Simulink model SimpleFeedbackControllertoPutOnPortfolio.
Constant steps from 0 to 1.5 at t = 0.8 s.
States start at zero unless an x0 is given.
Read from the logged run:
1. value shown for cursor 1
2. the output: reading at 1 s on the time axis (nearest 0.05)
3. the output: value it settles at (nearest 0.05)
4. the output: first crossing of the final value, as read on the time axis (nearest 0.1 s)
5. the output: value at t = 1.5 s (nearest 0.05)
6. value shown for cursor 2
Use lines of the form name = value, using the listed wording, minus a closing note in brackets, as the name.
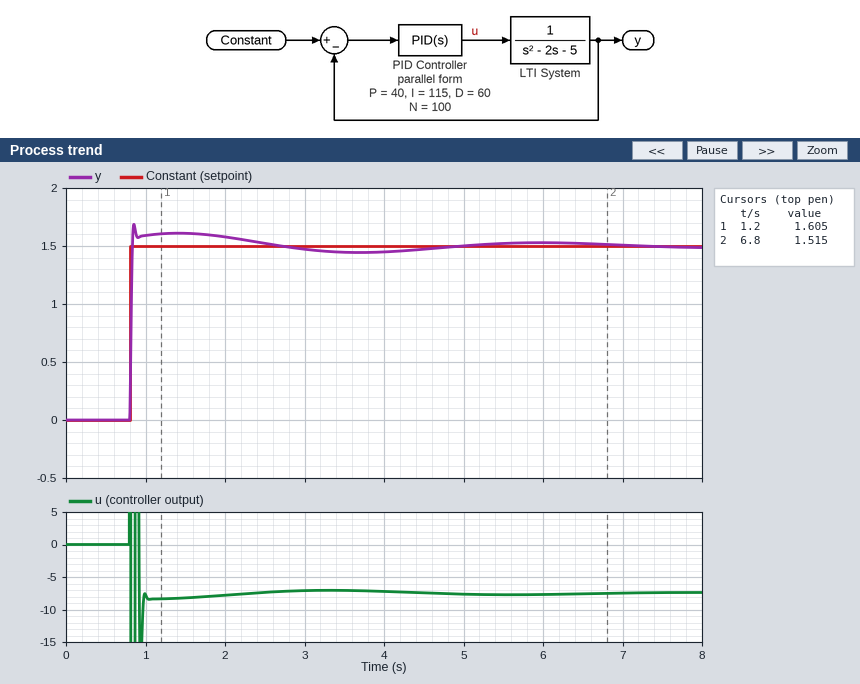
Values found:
value shown for cursor 1 = 1.605
the output: reading at 1 s on the time axis = 1.60
the output: value it settles at = 1.50
the output: first crossing of the final value, as read on the time axis = 0.8 s
the output: value at t = 1.5 s = 1.60
value shown for cursor 2 = 1.515
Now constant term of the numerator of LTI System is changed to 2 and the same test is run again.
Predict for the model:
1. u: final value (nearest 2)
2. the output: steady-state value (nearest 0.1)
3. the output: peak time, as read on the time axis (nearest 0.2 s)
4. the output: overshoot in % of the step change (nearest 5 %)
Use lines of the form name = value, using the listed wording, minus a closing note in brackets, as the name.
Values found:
u: final value = -4
the output: steady-state value = 1.5
the output: peak time, as read on the time axis = 0.8 s
the output: overshoot in % of the step change = 25 %
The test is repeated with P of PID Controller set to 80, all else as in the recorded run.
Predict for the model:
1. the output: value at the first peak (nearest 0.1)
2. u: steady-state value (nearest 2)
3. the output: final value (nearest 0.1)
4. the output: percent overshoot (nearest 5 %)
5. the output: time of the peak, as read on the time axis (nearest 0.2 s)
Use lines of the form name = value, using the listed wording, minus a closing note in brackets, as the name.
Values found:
the output: value at the first peak = 1.7
u: steady-state value = -8
the output: final value = 1.5
the output: percent overshoot = 15 %
the output: time of the peak, as read on the time axis = 0.8 s
